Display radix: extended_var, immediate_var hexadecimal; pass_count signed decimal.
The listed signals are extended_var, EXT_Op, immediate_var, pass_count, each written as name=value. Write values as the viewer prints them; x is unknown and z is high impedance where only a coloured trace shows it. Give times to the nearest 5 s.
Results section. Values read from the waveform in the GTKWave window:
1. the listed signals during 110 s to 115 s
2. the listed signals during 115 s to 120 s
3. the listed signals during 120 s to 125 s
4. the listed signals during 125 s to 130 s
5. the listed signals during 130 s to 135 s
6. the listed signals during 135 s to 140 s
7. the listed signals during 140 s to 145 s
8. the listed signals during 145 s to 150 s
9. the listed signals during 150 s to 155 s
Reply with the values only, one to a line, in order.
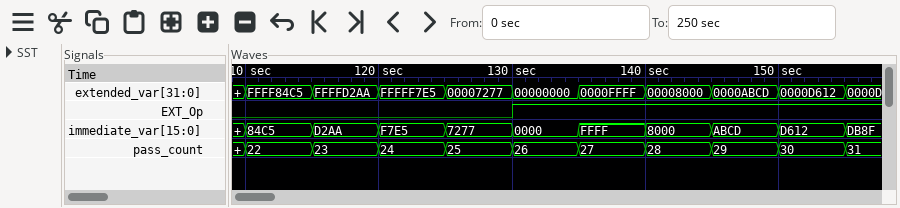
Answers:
extended_var=FFFF84C5, EXT_Op=0, immediate_var=84C5, pass_count=22
extended_var=FFFFD2AA, EXT_Op=0, immediate_var=D2AA, pass_count=23
extended_var=FFFFF7E5, EXT_Op=0, immediate_var=F7E5, pass_count=24
extended_var=00007277, EXT_Op=0, immediate_var=7277, pass_count=25
extended_var=00000000, EXT_Op=1, immediate_var=0000, pass_count=26
extended_var=0000FFFF, EXT_Op=1, immediate_var=FFFF, pass_count=27
extended_var=00008000, EXT_Op=1, immediate_var=8000, pass_count=28
extended_var=0000ABCD, EXT_Op=1, immediate_var=ABCD, pass_count=29
extended_var=0000D612, EXT_Op=1, immediate_var=D612, pass_count=30
